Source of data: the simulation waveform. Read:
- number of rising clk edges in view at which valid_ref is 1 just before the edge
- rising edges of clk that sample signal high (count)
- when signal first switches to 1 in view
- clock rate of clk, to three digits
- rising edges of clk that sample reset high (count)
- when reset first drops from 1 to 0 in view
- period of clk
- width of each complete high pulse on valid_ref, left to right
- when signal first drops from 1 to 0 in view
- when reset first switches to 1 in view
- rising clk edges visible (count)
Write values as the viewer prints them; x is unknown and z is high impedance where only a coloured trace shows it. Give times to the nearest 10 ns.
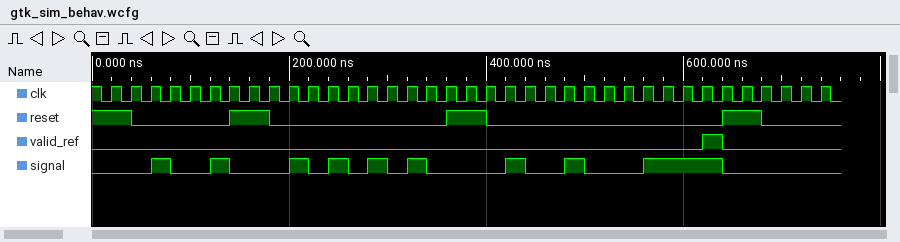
1
12
60 ns
50.0 MHz
8
40 ns
20 ns
20 ns
80 ns
140 ns
37
